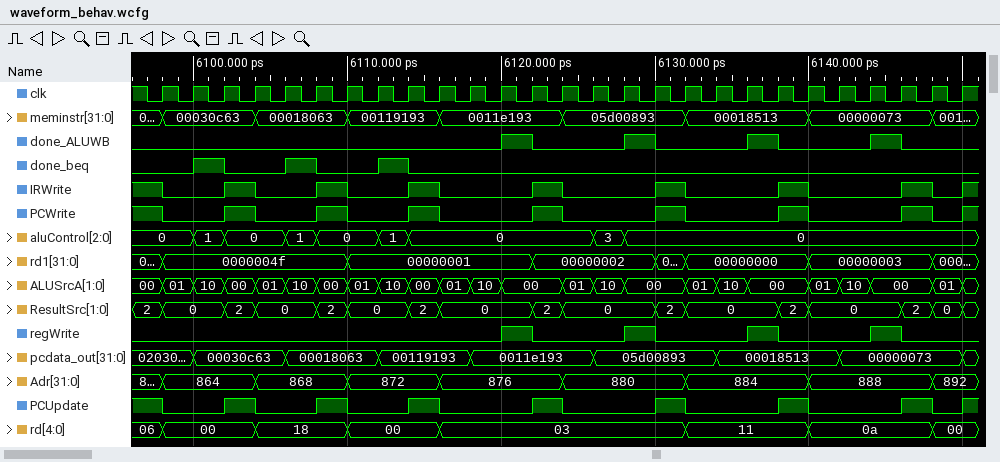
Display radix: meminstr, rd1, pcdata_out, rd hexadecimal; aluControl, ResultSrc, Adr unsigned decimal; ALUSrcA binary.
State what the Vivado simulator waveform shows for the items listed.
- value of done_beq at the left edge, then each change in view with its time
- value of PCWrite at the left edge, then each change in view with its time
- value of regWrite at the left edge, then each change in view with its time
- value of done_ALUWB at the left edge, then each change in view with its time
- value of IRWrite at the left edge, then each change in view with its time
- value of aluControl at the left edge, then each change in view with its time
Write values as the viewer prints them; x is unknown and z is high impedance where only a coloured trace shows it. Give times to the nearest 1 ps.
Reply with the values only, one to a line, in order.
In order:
0, 1 at 6100 ps, 0 at 6102 ps, 1 at 6106 ps, 0 at 6108 ps, 1 at 6112 ps, 0 at 6114 ps
1, 0 at 6098 ps, 1 at 6102 ps, 0 at 6104 ps, 1 at 6108 ps, 0 at 6110 ps, 1 at 6114 ps, 0 at 6116 ps, 1 at 6122 ps, 0 at 6124 ps, 1 at 6130 ps, 0 at 6132 ps, 1 at 6138 ps, 0 at 6140 ps, 1 at 6146 ps, 0 at 6148 ps, 1 at 6150 ps
0, 1 at 6120 ps, 0 at 6122 ps, 1 at 6128 ps, 0 at 6130 ps, 1 at 6136 ps, 0 at 6138 ps, 1 at 6144 ps, 0 at 6146 ps
0, 1 at 6120 ps, 0 at 6122 ps, 1 at 6128 ps, 0 at 6130 ps, 1 at 6136 ps, 0 at 6138 ps, 1 at 6144 ps, 0 at 6146 ps
1, 0 at 6098 ps, 1 at 6102 ps, 0 at 6104 ps, 1 at 6108 ps, 0 at 6110 ps, 1 at 6114 ps, 0 at 6116 ps, 1 at 6122 ps, 0 at 6124 ps, 1 at 6130 ps, 0 at 6132 ps, 1 at 6138 ps, 0 at 6140 ps, 1 at 6146 ps, 0 at 6148 ps, 1 at 6150 ps
0, 1 at 6100 ps, 0 at 6102 ps, 1 at 6106 ps, 0 at 6108 ps, 1 at 6112 ps, 0 at 6114 ps, 3 at 6126 ps, 0 at 6128 ps
